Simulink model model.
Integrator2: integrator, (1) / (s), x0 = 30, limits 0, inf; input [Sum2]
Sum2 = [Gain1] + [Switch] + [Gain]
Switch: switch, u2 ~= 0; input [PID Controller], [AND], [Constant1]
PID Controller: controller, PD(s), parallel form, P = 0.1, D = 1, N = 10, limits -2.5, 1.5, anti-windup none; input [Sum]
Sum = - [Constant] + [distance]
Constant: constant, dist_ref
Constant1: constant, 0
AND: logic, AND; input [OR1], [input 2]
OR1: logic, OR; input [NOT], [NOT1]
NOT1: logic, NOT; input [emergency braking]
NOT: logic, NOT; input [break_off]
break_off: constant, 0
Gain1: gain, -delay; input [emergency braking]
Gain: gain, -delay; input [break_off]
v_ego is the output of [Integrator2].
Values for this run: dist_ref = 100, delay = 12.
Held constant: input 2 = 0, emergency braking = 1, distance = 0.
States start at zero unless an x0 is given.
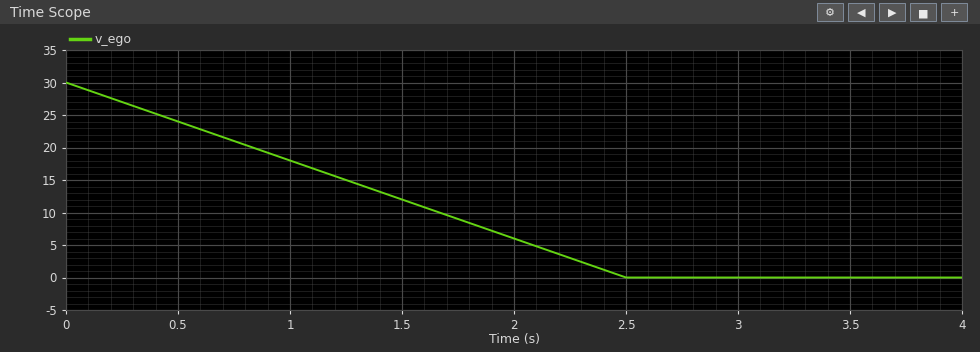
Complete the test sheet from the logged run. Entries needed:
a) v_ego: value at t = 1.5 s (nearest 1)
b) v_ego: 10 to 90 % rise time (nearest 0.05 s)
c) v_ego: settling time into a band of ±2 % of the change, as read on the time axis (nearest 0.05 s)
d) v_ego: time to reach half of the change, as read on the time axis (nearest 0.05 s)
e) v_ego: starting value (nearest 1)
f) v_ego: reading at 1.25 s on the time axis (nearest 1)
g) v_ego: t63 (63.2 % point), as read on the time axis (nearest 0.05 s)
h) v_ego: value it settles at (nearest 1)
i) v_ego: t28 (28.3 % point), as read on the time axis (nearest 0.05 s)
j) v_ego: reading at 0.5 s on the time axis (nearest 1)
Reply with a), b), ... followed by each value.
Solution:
a) 12
b) 2.00 s
c) 2.45 s
d) 1.25 s
e) 30
f) 15
g) 1.60 s
h) 0
i) 0.70 s
j) 24
